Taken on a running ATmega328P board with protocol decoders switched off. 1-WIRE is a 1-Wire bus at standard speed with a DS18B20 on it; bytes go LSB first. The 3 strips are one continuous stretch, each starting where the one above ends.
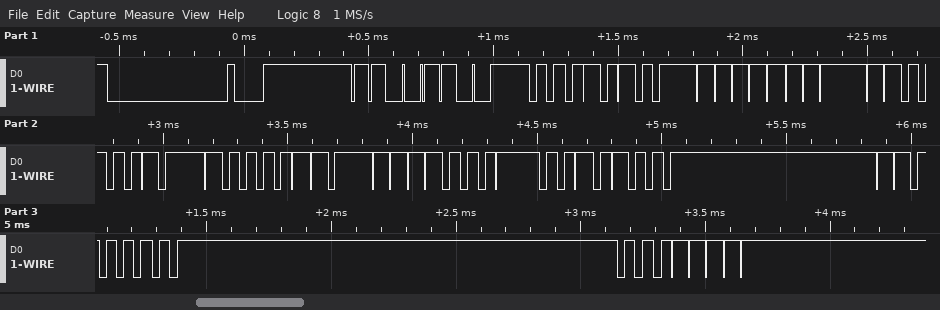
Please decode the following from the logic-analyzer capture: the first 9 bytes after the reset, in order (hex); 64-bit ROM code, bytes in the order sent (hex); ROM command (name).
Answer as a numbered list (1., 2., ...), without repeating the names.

1. 33 28 FF 43 61 8F 14 03 F8
2. 28 FF 43 61 8F 14 03 F8
3. Read ROM
